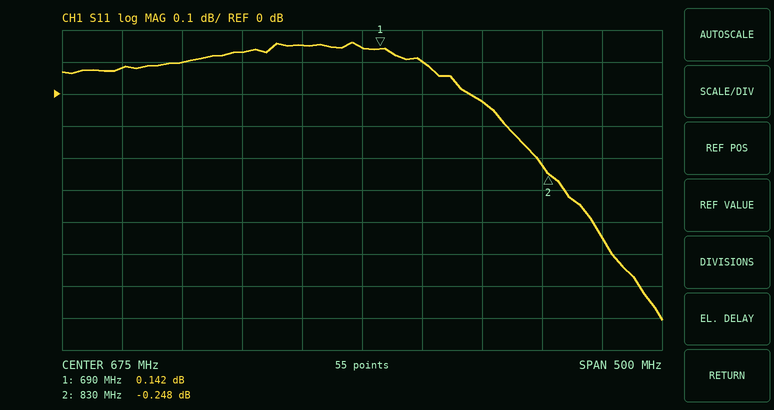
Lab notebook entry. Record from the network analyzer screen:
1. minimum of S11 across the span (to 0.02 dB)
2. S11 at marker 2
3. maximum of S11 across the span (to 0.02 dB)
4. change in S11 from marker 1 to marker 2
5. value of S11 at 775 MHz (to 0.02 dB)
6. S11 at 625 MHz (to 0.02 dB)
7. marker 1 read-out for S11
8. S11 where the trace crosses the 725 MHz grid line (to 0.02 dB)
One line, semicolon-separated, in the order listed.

-0.70 dB; -0.248 dB; 0.16 dB; -0.390 dB; -0.02 dB; 0.16 dB; 0.142 dB; 0.10 dB
